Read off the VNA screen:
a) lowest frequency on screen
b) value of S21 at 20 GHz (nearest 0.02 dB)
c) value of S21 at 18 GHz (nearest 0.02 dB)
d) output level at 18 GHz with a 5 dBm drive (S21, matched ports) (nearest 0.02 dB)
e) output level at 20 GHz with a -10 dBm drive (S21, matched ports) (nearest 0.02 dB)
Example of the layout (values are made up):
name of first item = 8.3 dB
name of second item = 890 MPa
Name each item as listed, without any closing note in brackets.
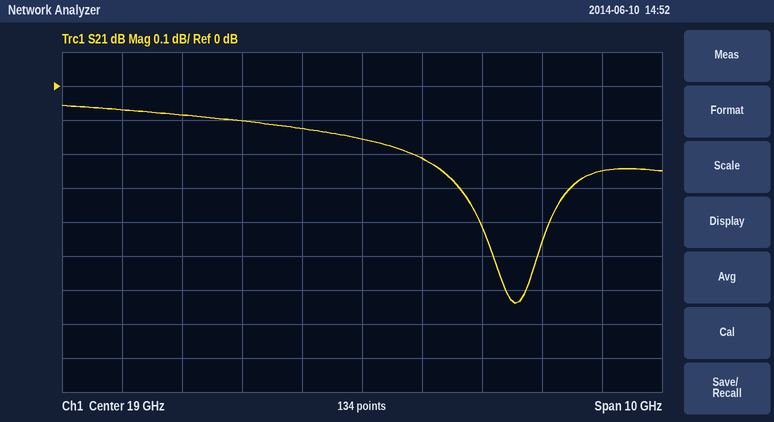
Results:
lowest frequency on screen = 14 GHz
value of S21 at 20 GHz = -0.22 dB
value of S21 at 18 GHz = -0.12 dB
output level at 18 GHz with a 5 dBm drive (S21, matched ports) = 4.88 dBm
output level at 20 GHz with a -10 dBm drive (S21, matched ports) = -10.22 dBm
